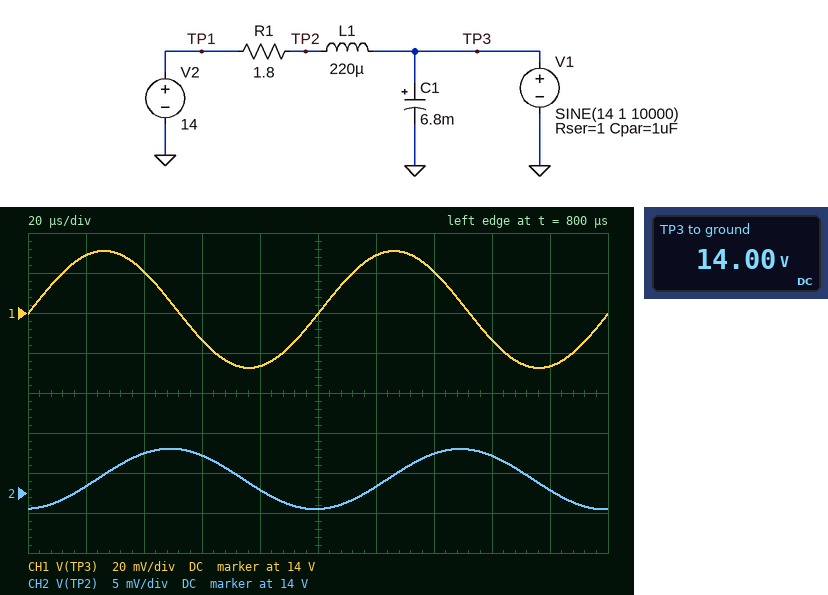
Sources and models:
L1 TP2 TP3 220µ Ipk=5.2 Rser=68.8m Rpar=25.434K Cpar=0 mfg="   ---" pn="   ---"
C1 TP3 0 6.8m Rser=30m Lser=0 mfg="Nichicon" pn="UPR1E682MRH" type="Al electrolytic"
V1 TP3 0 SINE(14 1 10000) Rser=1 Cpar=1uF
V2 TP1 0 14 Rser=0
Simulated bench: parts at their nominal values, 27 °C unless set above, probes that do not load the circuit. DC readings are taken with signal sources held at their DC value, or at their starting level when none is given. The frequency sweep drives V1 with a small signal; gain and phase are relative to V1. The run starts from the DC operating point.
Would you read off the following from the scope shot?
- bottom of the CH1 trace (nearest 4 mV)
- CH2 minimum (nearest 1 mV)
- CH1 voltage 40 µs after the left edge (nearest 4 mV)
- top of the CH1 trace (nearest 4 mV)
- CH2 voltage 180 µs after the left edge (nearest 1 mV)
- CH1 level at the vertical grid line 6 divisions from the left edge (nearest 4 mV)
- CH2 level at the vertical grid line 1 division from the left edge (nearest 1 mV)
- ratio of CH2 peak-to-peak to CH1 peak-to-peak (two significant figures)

13.972 V
13.998 V
14.020 V
14.032 V
14.000 V
14.028 V
14.001 V
0.13
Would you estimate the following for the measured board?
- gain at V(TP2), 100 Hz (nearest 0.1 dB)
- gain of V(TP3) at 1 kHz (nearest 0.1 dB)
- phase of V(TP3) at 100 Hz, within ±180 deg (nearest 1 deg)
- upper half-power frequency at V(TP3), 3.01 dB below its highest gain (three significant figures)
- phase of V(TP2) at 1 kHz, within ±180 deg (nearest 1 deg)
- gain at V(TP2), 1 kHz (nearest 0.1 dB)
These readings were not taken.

-13.7 dB
-28.7 dB
-64 deg
34.7 Hz
-72 deg
-30.9 dB
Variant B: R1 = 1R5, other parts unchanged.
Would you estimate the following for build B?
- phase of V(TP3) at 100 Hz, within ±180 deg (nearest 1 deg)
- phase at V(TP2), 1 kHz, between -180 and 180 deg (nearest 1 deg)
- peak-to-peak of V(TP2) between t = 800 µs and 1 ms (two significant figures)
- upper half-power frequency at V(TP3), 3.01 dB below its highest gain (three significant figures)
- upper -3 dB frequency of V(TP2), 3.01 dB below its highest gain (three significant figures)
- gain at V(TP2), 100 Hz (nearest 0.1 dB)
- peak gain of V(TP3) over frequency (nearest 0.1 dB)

-62 deg
-77 deg
6.4 mV
37.1 Hz
37.0 Hz
-13.8 dB
-4.3 dB
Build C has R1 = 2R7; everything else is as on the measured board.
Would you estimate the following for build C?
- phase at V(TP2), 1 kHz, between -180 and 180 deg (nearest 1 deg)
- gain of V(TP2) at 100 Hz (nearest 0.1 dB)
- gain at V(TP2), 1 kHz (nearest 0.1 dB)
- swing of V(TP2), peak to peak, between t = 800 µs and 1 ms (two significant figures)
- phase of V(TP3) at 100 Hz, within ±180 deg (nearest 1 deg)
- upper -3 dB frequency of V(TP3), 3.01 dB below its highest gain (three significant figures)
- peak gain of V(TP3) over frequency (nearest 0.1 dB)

-63 deg
-13.5 dB
-29.9 dB
11 mV
-66 deg
30.8 Hz
-2.7 dB
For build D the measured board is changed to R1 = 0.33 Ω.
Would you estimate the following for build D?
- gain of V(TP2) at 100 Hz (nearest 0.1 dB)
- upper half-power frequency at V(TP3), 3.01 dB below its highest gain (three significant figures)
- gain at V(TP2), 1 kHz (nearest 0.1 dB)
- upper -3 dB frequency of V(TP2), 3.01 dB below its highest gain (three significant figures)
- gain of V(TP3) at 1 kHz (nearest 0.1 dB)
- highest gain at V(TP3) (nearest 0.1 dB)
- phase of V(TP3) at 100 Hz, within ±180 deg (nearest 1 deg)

-16.3 dB
94.8 Hz
-41.4 dB
86.8 Hz
-28.6 dB
-10.9 dB
-42 deg
